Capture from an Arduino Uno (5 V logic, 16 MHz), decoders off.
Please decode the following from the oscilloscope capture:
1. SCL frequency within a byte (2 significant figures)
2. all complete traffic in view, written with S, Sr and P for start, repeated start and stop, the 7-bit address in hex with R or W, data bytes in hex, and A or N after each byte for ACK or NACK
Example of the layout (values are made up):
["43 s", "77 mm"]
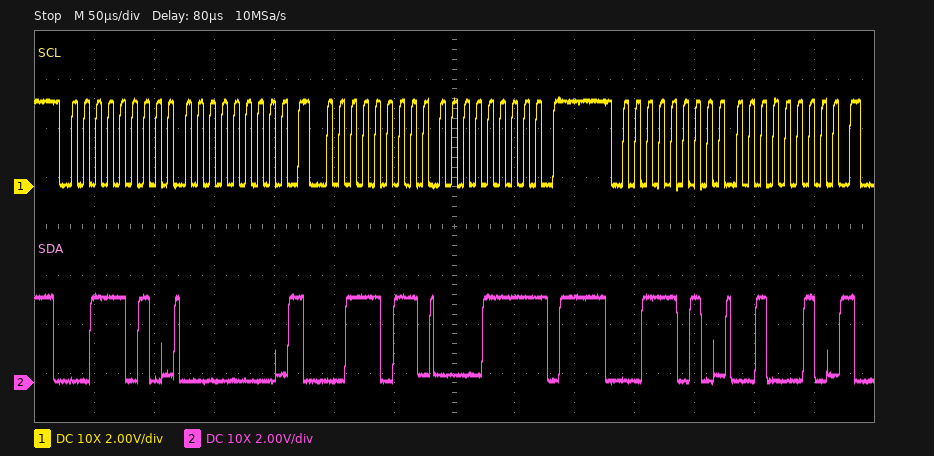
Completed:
["100 kHz", "S 1DW A 00 A Sr 1DR A 0F N P S 1DW A 22 A"]
